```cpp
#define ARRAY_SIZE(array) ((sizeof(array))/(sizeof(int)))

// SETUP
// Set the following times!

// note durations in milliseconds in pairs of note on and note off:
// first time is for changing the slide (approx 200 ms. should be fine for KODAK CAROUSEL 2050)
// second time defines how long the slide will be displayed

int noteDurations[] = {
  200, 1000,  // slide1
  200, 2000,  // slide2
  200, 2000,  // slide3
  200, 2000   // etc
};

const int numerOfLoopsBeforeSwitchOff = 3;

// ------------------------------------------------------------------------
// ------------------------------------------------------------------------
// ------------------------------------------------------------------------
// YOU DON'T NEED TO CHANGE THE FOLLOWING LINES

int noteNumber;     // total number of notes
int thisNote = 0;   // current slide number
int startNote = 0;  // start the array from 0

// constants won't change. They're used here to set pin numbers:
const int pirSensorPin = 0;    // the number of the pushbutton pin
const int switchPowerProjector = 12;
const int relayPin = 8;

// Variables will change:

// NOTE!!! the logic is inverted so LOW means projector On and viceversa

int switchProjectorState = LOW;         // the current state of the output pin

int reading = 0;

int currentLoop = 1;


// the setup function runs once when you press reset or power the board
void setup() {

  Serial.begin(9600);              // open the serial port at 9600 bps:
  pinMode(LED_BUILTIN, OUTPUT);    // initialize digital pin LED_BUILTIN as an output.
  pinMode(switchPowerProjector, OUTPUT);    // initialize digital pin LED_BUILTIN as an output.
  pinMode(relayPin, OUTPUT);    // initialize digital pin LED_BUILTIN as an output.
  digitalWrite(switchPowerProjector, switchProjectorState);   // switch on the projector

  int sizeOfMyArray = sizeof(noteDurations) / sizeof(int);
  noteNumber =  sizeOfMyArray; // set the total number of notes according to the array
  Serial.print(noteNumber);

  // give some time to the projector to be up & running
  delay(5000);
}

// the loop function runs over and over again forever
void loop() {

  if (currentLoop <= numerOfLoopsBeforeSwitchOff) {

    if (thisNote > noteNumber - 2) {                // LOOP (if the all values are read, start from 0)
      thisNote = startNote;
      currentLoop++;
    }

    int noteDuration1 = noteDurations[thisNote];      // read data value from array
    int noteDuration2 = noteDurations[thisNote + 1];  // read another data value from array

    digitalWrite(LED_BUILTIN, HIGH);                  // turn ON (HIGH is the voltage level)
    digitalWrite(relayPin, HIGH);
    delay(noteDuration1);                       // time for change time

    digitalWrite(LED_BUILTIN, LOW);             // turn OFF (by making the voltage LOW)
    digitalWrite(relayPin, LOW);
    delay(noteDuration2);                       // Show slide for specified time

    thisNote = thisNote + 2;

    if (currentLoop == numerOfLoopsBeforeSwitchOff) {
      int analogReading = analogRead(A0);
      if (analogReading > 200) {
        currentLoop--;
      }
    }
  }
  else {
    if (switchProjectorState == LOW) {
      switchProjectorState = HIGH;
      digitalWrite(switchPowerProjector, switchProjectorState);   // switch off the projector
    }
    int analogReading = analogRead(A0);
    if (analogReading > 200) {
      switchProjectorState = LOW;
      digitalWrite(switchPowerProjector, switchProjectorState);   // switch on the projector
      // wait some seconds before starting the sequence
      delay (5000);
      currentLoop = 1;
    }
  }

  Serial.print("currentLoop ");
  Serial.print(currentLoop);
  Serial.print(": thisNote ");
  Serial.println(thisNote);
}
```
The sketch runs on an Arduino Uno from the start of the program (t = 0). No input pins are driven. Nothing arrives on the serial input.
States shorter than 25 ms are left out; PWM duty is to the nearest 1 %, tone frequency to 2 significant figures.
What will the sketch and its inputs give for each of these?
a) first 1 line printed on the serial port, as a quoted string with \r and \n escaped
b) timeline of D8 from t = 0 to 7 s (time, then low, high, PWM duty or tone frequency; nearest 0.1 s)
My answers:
"8currentLoop 1: thisNote 2\r\n"
0 s low; 5 s high; 5.2 s low; 6.2 s high; 6.4 s low
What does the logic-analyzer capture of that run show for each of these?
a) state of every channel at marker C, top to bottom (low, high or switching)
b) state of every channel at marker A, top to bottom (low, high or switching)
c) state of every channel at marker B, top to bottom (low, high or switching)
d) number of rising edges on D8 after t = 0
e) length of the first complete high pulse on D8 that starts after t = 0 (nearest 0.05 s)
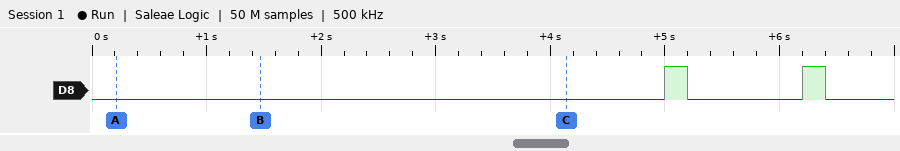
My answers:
D8 low
D8 low
D8 low
2
0.20 s
